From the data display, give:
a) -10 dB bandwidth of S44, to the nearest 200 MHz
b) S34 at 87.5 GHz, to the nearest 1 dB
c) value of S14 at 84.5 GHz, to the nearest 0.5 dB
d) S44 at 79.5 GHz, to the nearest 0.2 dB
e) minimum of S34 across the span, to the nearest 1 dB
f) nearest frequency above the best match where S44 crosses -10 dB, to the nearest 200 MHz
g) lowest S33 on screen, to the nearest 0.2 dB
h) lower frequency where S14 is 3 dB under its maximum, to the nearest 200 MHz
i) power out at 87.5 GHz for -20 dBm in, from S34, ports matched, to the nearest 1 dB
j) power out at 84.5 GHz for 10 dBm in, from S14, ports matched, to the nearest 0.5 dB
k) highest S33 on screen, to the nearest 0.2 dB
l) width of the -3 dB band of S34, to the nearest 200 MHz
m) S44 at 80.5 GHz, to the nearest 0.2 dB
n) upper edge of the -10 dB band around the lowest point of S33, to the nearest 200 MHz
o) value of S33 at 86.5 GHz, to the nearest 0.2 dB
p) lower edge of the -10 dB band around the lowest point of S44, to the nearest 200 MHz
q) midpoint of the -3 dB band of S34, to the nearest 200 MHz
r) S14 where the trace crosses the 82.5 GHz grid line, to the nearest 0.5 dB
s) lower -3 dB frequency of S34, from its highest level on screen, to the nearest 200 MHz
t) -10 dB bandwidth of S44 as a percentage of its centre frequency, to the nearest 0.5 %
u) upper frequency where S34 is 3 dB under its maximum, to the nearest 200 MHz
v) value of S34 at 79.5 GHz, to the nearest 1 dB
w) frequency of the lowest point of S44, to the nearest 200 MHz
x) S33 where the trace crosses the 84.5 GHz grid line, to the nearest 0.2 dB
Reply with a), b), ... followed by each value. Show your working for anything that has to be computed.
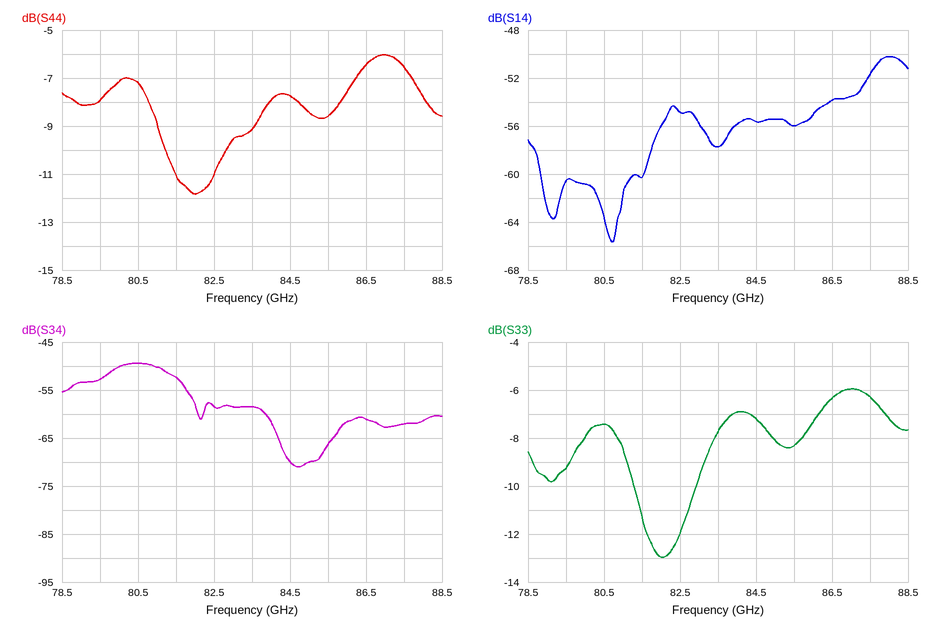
a) 82.8 GHz − 81.2 GHz = 1.6 GHz
b) -62 dB
c) -55.5 dB
d) -8.0 dB
e) -71 dB
f) 82.8 GHz
g) -13.0 dB
h) 87.2 GHz
i) -20 dBm + (-62 dB) = -82 dBm
j) 10 dBm + (-55.5 dB) = -45.5 dBm
k) -6.0 dB
l) 81.6 GHz − 79.6 GHz = 2.0 GHz
m) -7.2 dB
n) 83.0 GHz
o) -6.4 dB
p) 81.2 GHz
q) 80.6 GHz
r) -55.0 dB
s) 79.6 GHz
t) 1.6 GHz / 82 GHz ≈ 2.0 %
u) 81.6 GHz
v) -53 dB
w) 82.0 GHz
x) -7.2 dB
